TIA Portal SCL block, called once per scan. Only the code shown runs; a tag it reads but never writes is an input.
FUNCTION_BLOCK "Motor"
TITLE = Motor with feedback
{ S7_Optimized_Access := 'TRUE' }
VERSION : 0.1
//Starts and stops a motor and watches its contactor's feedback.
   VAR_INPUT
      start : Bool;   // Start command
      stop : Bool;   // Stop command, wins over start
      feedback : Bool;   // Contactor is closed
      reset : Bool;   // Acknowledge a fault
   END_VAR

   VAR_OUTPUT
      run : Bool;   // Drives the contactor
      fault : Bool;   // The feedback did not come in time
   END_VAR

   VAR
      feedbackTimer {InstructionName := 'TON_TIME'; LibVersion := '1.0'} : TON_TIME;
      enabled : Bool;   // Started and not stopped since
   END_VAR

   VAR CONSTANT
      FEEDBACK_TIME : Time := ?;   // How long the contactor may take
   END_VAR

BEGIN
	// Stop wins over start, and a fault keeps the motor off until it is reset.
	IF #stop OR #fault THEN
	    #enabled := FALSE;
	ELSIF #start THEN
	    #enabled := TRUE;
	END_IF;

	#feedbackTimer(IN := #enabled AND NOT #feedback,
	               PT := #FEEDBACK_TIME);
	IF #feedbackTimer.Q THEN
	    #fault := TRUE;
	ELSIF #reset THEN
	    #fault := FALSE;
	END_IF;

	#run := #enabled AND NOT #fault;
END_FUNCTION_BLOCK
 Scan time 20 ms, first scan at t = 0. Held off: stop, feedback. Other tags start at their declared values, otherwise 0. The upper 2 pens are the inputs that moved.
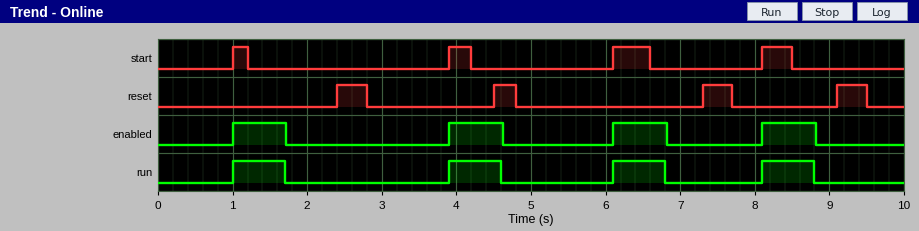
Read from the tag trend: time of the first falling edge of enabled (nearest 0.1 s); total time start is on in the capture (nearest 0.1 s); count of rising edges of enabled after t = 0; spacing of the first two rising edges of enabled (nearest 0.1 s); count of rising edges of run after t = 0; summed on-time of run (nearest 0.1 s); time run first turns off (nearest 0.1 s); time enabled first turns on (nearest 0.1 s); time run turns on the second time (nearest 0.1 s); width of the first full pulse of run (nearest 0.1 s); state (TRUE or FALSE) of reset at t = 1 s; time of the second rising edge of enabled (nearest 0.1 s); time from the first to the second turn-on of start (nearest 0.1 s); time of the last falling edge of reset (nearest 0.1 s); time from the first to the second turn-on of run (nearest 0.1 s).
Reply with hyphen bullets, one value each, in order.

- 1.7 s
- 1.4 s
- 4
- 2.9 s
- 4
- 2.8 s
- 1.7 s
- 1.0 s
- 3.9 s
- 0.7 s
- FALSE
- 3.9 s
- 2.9 s
- 9.5 s
- 2.9 s
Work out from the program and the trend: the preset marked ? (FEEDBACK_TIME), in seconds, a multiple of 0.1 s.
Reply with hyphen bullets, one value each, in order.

- 0.7 s
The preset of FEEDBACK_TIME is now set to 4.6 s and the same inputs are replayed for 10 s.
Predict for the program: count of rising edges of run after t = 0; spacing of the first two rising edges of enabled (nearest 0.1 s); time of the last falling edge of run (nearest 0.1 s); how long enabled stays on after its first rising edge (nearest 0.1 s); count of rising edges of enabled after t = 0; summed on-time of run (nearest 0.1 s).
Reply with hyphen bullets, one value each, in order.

- 2
- 7.1 s
- 5.6 s
- 4.6 s
- 2
- 6.5 s
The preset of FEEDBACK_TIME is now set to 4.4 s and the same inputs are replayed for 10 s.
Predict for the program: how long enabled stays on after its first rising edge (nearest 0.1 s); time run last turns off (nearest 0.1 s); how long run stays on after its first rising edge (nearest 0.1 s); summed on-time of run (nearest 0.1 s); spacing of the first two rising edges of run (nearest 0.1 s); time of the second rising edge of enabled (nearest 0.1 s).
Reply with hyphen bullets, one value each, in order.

- 4.4 s
- 5.4 s
- 4.4 s
- 6.3 s
- 7.1 s
- 8.1 s
